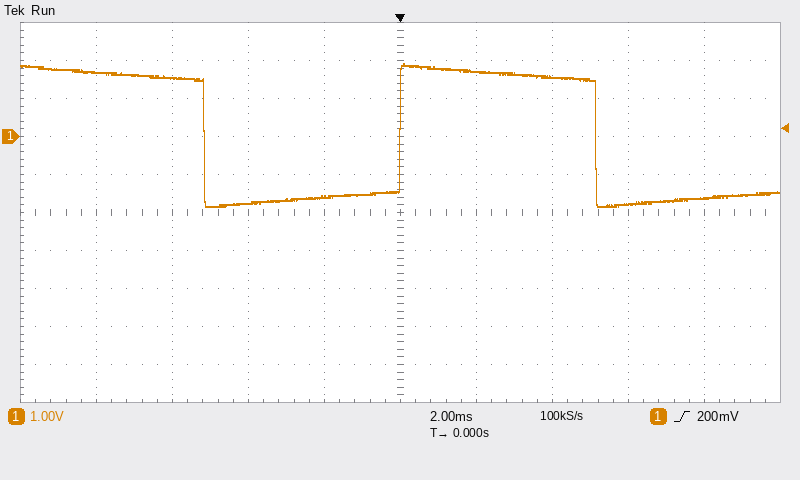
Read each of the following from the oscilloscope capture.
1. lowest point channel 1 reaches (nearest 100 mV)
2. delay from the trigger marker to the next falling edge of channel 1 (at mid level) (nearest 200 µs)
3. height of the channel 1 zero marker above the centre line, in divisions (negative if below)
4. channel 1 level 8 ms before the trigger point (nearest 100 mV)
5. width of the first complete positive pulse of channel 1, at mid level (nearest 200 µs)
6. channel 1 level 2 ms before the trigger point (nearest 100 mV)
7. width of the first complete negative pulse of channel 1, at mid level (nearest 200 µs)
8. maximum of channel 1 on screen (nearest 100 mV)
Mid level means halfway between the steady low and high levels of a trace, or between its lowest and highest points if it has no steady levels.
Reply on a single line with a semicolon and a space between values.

-1.8 V; 5.2 ms; +2.0 div; 1.7 V; 5.2 ms; -1.6 V; 5.2 ms; 1.9 V
